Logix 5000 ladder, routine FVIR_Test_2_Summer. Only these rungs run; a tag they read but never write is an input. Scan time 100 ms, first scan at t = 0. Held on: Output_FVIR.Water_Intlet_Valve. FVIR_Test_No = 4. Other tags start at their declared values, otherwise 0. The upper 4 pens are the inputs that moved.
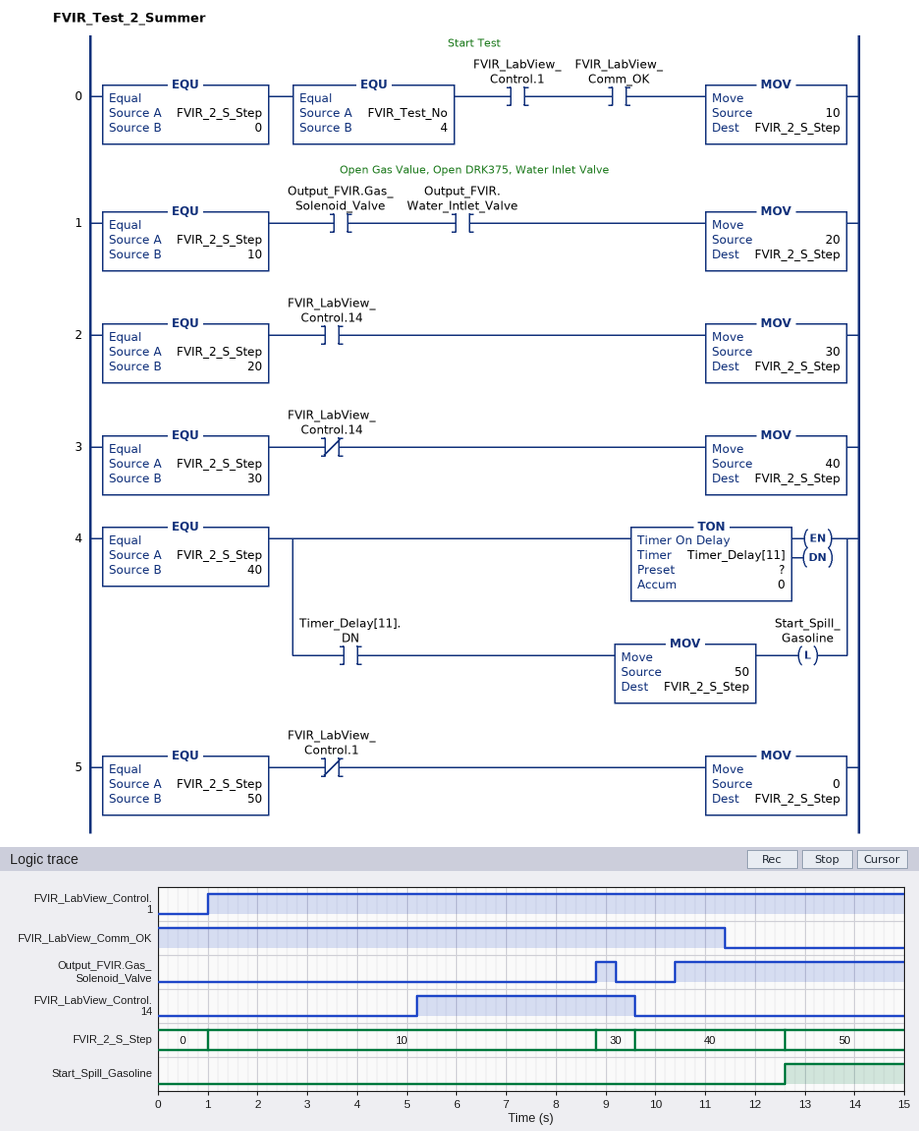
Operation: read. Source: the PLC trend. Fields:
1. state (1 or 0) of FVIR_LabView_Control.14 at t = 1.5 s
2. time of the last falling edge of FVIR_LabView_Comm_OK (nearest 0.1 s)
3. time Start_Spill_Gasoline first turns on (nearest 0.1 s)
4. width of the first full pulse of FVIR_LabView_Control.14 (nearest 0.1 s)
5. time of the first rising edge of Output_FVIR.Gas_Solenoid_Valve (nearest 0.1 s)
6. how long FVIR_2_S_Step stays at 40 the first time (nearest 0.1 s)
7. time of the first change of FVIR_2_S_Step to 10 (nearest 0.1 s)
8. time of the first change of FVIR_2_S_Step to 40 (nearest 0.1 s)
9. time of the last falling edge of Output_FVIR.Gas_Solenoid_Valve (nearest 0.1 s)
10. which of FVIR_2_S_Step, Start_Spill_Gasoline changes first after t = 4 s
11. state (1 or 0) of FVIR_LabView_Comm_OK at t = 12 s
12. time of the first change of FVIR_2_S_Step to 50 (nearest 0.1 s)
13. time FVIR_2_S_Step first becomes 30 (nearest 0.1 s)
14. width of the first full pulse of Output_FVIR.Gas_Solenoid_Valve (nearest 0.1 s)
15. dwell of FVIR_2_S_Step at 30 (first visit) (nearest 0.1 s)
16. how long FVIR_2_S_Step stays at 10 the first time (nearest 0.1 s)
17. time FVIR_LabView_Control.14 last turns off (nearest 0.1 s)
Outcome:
0
11.4 s
12.6 s
4.4 s
8.8 s
3.0 s
1.0 s
9.6 s
9.2 s
FVIR_2_S_Step
0
12.6 s
8.8 s
0.4 s
0.8 s
7.8 s
9.6 s
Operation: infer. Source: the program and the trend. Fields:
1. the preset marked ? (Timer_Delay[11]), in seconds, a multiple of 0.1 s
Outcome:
3.0 s
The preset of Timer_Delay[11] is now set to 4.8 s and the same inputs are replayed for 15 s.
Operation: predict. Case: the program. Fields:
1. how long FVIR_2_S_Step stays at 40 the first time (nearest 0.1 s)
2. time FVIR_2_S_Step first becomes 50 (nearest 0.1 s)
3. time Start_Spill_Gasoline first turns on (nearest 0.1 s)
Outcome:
4.8 s
14.4 s
14.4 s
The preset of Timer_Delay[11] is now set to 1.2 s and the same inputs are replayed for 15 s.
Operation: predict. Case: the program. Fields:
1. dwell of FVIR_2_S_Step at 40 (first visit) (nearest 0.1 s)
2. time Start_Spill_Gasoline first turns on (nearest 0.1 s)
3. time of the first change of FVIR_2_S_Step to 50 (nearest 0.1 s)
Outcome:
1.2 s
10.8 s
10.8 s
